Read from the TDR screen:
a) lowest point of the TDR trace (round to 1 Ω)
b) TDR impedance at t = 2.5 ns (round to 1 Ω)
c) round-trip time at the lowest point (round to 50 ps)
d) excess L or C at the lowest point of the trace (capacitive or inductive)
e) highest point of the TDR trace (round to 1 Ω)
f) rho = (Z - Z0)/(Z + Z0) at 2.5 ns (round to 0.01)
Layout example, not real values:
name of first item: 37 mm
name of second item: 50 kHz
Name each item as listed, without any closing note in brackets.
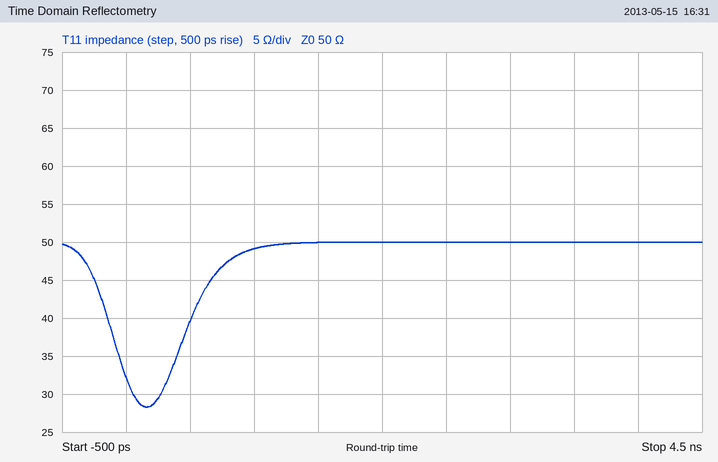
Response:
lowest point of the TDR trace: 28 Ω
TDR impedance at t = 2.5 ns: 50 Ω
round-trip time at the lowest point: 150 ps
excess L or C at the lowest point of the trace: capacitive
highest point of the TDR trace: 50 Ω
rho = (Z - Z0)/(Z + Z0) at 2.5 ns: 0.00
